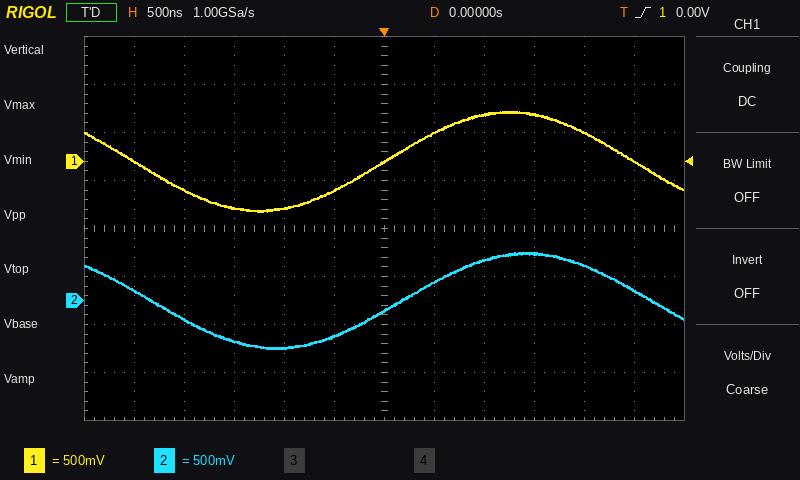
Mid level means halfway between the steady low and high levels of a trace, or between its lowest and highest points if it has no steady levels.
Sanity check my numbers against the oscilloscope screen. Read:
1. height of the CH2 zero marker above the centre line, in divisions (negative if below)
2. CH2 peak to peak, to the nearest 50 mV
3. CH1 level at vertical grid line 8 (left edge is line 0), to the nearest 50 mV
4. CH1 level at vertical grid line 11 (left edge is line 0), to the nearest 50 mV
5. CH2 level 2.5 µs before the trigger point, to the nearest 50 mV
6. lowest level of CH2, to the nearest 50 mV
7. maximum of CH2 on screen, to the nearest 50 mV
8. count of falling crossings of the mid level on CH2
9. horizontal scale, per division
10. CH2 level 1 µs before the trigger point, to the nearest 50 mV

-1.5 div
1.00 V
500 mV
0 mV
100 mV
-500 mV
500 mV
2
500 ns
-500 mV
